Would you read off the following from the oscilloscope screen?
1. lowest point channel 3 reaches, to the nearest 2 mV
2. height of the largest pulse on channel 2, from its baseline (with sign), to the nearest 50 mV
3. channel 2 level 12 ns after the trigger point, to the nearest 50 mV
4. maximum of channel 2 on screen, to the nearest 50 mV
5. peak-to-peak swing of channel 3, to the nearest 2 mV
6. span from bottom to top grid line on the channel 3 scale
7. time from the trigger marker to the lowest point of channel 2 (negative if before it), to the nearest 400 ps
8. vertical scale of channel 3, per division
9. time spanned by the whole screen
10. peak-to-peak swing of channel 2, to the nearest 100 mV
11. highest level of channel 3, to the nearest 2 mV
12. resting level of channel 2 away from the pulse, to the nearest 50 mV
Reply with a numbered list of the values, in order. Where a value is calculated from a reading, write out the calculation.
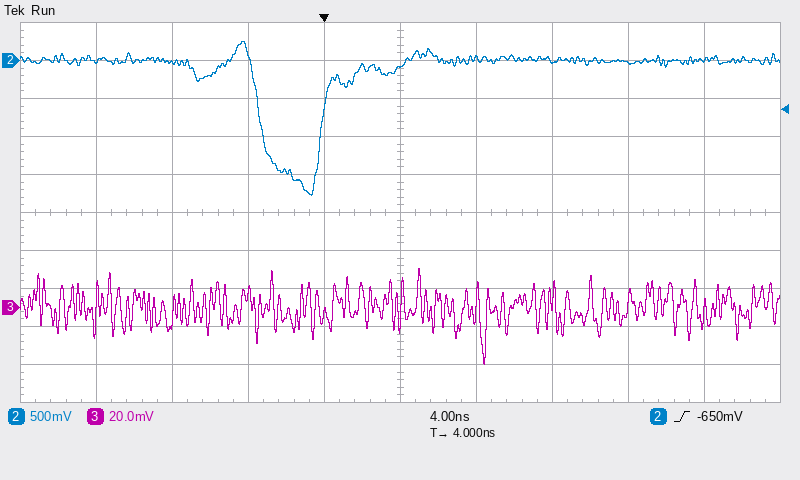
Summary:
1. -30 mV
2. -1.75 V
3. 0 mV
4. 250 mV
5. 20 mV − (-30 mV) = 50 mV
6. 200 mV
7. -800 ps
8. 20 mV
9. 40 ns
10. 2.00 V
11. 20 mV
12. 0 mV
